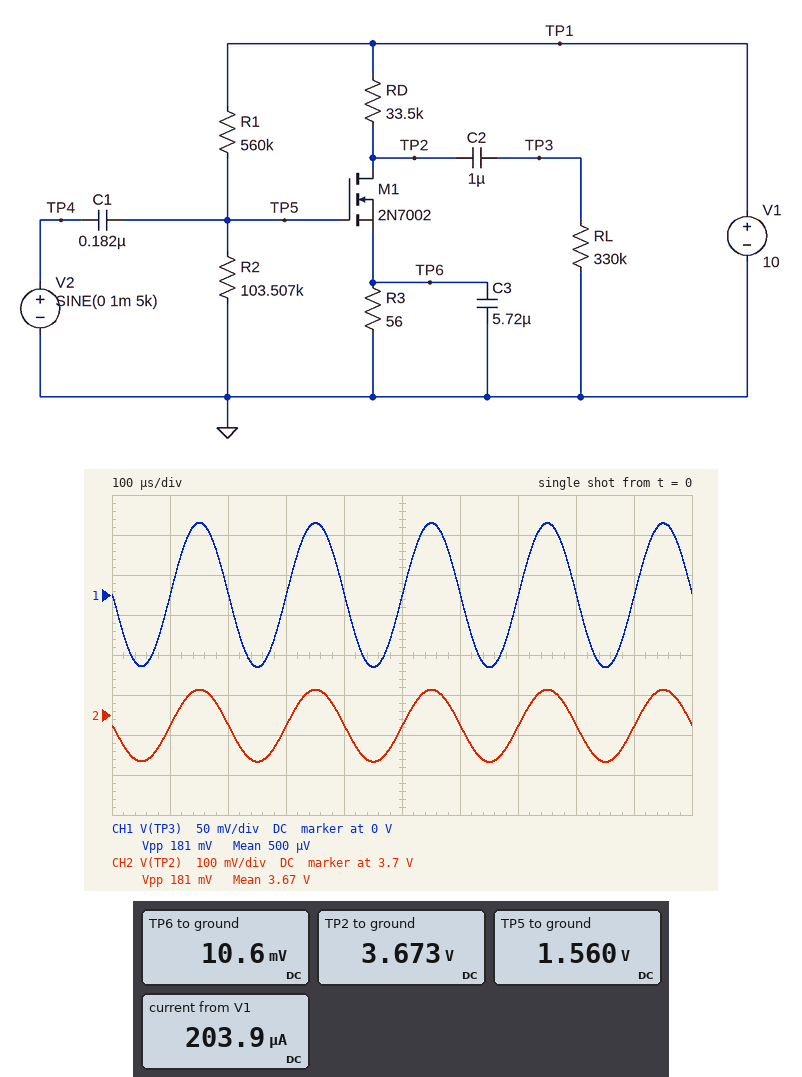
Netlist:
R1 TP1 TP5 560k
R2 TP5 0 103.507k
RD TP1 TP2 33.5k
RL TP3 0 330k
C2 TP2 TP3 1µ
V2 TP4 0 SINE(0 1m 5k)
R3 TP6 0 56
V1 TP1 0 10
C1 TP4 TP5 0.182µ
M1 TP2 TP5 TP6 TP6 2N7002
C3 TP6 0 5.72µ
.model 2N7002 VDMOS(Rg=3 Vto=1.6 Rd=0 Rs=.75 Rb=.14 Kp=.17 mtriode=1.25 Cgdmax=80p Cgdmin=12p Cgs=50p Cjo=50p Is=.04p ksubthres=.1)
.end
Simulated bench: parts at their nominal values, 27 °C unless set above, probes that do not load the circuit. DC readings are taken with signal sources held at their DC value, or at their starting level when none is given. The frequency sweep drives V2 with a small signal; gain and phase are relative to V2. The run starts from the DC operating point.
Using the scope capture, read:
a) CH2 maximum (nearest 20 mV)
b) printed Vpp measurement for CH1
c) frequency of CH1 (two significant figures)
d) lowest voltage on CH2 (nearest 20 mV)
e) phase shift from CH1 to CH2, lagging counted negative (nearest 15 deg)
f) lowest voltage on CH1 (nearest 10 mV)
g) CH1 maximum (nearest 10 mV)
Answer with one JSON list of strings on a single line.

["3.76 V", "181 mV", "5.0 kHz", "3.58 V", "0 deg", "-90 mV", "90 mV"]
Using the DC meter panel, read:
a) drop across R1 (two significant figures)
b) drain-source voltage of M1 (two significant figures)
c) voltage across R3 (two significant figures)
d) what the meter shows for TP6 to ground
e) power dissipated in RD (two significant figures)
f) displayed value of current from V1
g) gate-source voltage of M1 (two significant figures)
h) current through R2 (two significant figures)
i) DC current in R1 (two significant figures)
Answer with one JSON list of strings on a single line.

["8.4 V", "3.7 V", "11 mV", "10.6 mV", "1.2 mW", "203.9 µA", "1.5 V", "15 µA", "15 µA"]
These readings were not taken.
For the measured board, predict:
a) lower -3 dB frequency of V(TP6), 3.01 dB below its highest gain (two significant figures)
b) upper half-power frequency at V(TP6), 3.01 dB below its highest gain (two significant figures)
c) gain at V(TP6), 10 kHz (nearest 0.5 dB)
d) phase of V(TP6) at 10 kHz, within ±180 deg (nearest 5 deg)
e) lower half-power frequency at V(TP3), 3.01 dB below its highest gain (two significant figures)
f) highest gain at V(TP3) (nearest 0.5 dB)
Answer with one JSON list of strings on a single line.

["9.6 Hz", "600 Hz", "-41.5 dB", "-90 deg", "14 Hz", "39.0 dB"]
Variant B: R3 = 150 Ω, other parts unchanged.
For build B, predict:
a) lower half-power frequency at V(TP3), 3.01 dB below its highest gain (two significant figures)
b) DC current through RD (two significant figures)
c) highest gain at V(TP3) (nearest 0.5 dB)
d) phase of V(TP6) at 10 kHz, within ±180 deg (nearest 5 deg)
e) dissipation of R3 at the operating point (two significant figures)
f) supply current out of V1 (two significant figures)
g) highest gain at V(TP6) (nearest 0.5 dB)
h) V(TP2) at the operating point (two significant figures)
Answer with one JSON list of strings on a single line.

["35 Hz", "150 µA", "37.5 dB", "-90 deg", "3.6 µW", "170 µA", "-11.5 dB", "4.8 V"]
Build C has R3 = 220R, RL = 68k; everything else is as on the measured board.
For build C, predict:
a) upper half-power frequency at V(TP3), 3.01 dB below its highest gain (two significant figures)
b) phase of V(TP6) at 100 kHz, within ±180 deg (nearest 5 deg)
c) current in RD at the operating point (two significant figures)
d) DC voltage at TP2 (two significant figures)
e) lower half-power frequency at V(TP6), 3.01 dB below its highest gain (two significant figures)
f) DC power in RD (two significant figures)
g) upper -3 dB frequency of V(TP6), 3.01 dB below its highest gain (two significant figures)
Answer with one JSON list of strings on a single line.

["190 kHz", "-100 deg", "140 µA", "5.4 V", "9.1 Hz", "630 µW", "210 Hz"]
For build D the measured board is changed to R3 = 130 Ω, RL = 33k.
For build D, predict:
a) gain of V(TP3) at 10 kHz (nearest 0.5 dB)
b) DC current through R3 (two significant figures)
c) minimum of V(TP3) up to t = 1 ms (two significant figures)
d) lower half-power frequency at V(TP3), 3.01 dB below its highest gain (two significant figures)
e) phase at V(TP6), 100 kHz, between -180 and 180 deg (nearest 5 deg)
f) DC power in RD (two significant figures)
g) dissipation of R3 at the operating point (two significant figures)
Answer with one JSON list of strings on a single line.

["32.5 dB", "160 µA", "-43 mV", "28 Hz", "-100 deg", "860 µW", "3.3 µW"]
